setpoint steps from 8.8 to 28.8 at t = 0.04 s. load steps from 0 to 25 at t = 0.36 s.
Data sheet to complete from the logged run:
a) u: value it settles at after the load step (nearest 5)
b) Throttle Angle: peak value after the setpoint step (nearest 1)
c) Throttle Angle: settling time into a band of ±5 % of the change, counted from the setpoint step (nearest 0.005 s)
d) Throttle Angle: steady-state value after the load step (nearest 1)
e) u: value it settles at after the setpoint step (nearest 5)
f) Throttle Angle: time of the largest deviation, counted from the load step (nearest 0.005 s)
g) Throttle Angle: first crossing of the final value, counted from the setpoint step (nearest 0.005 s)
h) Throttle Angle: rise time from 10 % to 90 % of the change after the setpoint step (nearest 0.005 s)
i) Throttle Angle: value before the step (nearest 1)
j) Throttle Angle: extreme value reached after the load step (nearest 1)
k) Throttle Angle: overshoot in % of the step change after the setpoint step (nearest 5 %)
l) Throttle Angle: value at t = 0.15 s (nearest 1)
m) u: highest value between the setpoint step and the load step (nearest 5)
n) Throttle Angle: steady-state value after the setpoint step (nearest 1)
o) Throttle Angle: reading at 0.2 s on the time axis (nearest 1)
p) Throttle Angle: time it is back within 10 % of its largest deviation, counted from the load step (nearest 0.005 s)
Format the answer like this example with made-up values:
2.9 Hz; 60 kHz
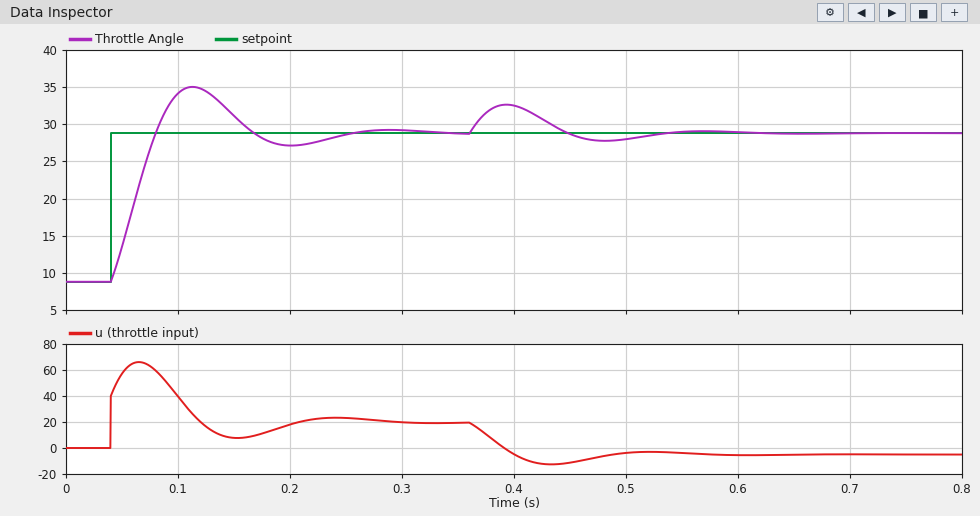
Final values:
-5; 35; 0.190 s; 29; 20; 0.035 s; 0.040 s; 0.030 s; 9; 33; 30 %; 31; 65; 29; 27; 0.160 s
